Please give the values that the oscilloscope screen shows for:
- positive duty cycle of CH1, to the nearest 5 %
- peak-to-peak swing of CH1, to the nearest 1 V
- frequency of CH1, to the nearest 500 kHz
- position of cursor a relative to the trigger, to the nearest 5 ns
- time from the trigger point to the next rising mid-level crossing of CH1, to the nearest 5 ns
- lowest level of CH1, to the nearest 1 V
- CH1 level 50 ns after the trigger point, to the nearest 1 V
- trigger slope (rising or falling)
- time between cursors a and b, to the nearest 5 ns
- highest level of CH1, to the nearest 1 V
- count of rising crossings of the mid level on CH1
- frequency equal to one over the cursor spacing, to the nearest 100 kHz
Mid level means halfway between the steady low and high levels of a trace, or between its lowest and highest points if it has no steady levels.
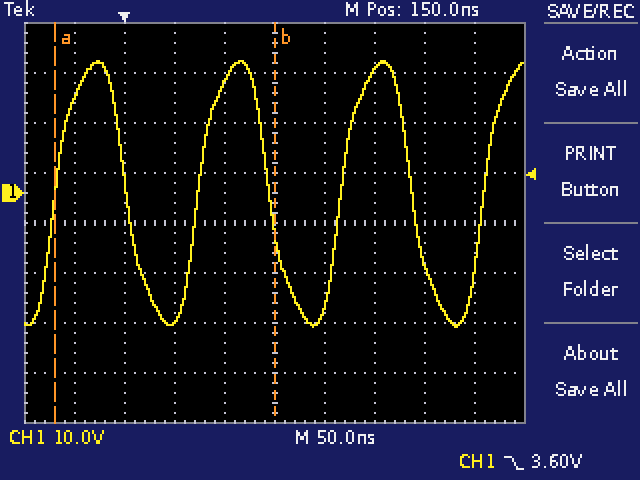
50 %
53 V
7.0 MHz
-70 ns
75 ns
-27 V
-26 V
falling
220 ns
26 V
4
4.5 MHz
